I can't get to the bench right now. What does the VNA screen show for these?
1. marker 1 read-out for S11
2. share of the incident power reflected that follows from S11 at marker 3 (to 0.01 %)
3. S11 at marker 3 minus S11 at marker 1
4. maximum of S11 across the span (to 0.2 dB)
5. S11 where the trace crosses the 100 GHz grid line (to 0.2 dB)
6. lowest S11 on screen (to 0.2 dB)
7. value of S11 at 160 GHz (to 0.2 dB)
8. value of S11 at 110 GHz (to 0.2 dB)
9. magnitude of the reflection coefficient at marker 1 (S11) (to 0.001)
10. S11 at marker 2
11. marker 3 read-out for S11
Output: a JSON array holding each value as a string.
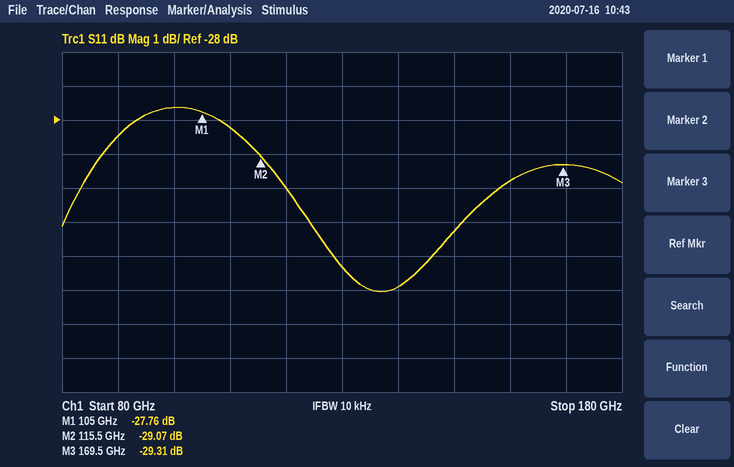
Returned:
["-27.76 dB", "0.12 %", "-1.55 dB", "-27.6 dB", "-27.6 dB", "-33.0 dB", "-29.8 dB", "-28.2 dB", "0.041", "-29.07 dB", "-29.31 dB"]
